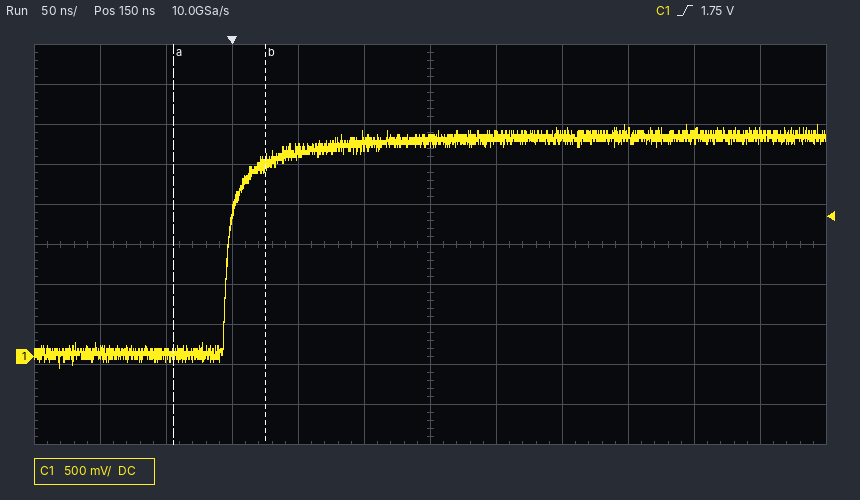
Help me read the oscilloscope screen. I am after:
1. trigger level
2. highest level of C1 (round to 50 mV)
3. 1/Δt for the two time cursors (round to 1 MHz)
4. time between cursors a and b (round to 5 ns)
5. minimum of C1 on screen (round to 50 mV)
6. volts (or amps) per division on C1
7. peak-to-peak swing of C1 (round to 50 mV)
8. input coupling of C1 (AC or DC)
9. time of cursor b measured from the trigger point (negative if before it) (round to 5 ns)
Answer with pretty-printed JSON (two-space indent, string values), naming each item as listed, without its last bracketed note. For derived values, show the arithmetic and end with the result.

{
  "trigger level": "1.75 V",
  "highest level of C1": "2.90 V",
  "1/Δt for the two time cursors": "1 / 70 ns ≈ 14 MHz",
  "time between cursors a and b": "70 ns",
  "minimum of C1 on screen": "-150 mV",
  "volts (or amps) per division on C1": "500 mV",
  "peak-to-peak swing of C1": "2.90 V − (-150 mV) = 3.05 V",
  "input coupling of C1": "DC",
  "time of cursor b measured from the trigger point (negative if before it)": "+25 ns"
}
